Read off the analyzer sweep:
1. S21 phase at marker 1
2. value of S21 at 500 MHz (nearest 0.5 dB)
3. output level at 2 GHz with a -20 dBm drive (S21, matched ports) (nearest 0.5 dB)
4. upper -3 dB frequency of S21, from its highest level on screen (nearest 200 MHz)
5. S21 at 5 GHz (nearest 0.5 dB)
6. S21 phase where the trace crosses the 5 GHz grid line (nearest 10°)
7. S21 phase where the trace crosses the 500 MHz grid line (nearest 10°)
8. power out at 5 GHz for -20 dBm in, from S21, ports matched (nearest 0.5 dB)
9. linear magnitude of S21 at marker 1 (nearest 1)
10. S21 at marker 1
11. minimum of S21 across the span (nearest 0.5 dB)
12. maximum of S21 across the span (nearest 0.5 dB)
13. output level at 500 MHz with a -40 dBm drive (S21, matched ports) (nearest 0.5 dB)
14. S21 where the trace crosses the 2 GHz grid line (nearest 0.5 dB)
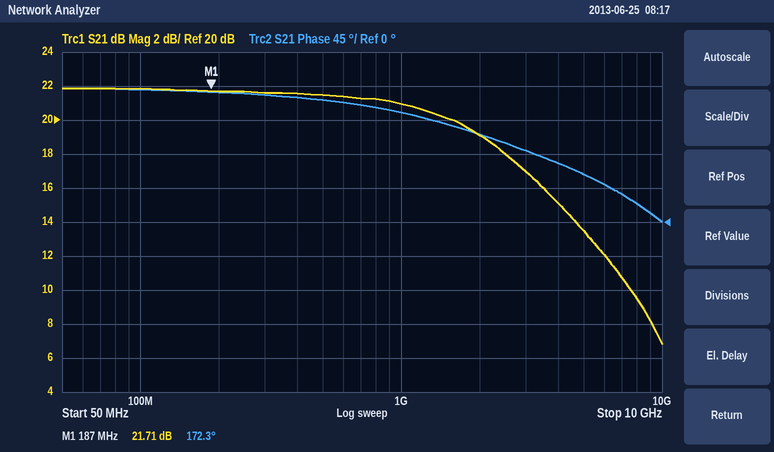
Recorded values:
172.3°
21.5 dB
-1.0 dBm
2.2 GHz
13.5 dB
60°
160°
-6.5 dBm
12
21.71 dB
7.0 dB
22.0 dB
-18.5 dBm
19.0 dB
